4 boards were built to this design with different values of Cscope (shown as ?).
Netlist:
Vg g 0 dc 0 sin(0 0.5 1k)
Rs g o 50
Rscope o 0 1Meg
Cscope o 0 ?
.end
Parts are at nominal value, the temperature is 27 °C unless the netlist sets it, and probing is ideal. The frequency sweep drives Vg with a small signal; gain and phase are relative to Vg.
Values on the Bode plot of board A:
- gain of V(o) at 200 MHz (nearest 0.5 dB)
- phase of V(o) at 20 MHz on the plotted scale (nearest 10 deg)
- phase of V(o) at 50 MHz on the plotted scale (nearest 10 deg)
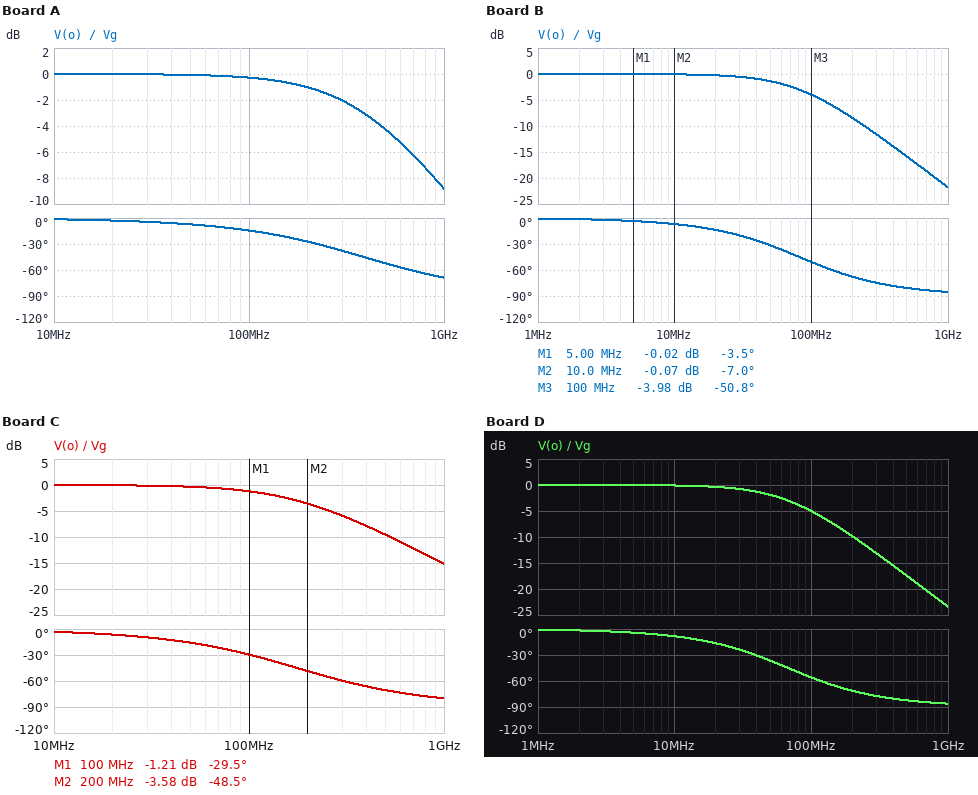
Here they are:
-1.0 dB
0 deg
-10 deg
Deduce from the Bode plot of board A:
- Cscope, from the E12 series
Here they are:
8.2 pF
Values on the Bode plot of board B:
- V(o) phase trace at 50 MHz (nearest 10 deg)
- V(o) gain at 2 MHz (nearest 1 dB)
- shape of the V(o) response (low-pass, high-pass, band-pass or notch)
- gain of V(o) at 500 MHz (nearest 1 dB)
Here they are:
-30 deg
0 dB
low-pass
-16 dB
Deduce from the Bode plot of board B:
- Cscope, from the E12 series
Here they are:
39 pF
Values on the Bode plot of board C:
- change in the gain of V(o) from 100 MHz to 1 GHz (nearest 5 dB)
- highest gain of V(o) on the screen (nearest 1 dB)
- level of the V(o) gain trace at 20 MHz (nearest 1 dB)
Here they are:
-15 dB
0 dB
0 dB
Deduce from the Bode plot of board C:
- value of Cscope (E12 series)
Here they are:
18 pF
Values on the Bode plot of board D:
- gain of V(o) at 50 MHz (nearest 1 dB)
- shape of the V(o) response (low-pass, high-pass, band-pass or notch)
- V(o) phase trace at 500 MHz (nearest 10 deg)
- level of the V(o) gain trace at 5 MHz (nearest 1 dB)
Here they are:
-2 dB
low-pass
-80 deg
0 dB
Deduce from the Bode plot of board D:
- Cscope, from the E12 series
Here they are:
47 pF
